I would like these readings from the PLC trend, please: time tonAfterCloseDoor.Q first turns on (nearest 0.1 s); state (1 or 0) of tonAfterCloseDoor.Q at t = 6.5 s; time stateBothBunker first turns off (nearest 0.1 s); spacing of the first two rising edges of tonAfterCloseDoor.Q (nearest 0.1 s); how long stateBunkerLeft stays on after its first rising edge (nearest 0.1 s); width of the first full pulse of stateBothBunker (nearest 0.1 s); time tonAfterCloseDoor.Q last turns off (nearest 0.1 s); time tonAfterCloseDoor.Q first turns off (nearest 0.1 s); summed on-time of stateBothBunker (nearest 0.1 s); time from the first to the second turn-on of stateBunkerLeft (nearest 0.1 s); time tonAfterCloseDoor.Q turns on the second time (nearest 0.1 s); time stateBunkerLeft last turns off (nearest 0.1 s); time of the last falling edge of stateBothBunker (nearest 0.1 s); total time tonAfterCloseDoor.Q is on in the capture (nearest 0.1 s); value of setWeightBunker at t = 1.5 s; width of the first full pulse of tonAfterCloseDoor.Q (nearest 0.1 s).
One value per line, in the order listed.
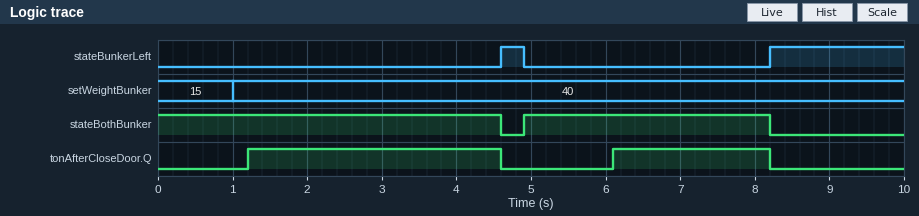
1.2 s
1
4.6 s
4.9 s
0.3 s
3.3 s
8.2 s
4.6 s
7.9 s
3.6 s
6.1 s
4.9 s
8.2 s
5.5 s
40
3.4 s
